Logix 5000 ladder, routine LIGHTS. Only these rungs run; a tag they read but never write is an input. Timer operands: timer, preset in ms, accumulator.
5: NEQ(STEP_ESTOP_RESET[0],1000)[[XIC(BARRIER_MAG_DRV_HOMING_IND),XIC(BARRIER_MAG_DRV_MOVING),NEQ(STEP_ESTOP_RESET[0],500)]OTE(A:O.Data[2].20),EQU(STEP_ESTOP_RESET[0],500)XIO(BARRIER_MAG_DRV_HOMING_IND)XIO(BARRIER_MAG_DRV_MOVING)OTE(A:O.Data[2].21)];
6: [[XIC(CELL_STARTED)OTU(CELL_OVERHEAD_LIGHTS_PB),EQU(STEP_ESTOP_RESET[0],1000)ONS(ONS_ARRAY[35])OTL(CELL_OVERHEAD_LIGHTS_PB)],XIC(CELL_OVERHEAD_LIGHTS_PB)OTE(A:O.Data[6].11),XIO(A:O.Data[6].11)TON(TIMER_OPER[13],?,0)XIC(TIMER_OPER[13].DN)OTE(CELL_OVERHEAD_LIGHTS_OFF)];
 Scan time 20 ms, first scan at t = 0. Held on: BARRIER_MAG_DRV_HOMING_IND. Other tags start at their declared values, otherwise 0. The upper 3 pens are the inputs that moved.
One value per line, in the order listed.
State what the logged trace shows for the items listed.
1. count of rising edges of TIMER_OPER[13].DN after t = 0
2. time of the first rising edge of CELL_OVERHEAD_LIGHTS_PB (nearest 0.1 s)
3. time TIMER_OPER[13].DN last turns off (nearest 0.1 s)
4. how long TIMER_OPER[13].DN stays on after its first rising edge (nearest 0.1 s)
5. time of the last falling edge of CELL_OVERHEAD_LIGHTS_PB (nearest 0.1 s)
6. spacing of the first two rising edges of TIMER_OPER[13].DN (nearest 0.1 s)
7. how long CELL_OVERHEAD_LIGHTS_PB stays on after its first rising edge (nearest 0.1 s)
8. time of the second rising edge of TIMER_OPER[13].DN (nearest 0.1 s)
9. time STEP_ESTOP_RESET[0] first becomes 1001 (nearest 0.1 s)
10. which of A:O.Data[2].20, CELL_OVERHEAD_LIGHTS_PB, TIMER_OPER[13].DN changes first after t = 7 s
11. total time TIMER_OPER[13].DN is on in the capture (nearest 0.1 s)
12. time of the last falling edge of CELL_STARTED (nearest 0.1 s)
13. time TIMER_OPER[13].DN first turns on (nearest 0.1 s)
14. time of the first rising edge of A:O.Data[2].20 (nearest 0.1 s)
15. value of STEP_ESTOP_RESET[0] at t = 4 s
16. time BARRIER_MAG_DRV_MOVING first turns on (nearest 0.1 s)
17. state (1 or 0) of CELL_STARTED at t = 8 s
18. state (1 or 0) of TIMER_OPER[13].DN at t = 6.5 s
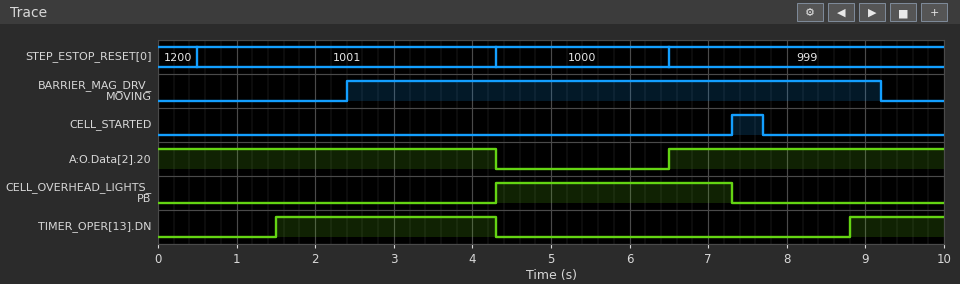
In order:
2
4.3 s
4.3 s
2.8 s
7.3 s
7.3 s
3.0 s
8.8 s
0.5 s
CELL_OVERHEAD_LIGHTS_PB
4.0 s
7.7 s
1.5 s
6.5 s
1001
2.4 s
0
0
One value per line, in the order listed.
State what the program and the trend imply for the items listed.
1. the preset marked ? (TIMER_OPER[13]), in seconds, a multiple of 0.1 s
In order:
1.5 s
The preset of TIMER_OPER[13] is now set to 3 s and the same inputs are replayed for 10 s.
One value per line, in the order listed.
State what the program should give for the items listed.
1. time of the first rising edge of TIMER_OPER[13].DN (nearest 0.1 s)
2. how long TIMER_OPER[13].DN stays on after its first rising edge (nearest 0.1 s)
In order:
3.0 s
1.3 s
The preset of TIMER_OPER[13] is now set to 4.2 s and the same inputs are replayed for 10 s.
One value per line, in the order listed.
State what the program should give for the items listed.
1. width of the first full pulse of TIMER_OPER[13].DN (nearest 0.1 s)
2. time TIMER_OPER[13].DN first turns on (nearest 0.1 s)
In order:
0.1 s
4.2 s
